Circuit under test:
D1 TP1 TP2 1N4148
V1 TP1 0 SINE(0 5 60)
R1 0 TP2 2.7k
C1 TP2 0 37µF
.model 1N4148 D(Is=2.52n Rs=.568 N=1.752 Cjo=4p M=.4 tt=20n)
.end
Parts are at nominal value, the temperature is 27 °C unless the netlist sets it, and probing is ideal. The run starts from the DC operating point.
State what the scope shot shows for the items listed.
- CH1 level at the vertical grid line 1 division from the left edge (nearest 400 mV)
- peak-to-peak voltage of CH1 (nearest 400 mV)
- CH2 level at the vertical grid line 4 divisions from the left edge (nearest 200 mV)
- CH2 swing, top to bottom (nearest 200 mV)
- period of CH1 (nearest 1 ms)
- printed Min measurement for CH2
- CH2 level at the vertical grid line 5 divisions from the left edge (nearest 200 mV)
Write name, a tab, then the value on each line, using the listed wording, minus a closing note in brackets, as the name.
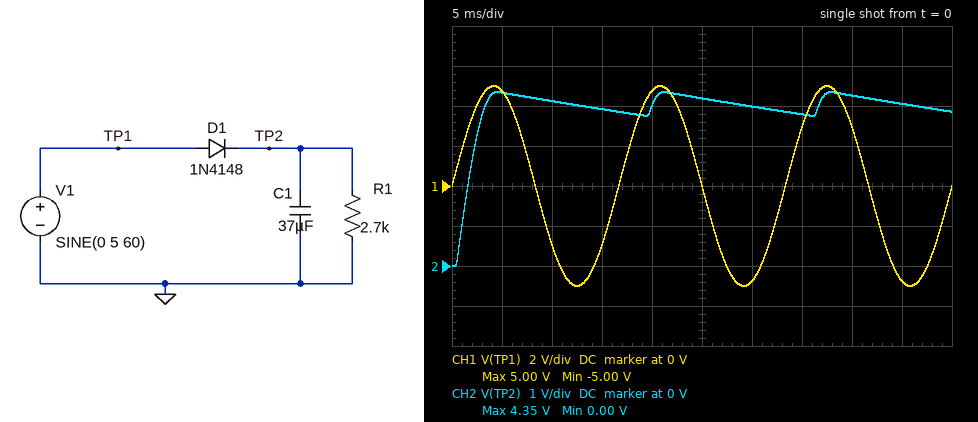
CH1 level at the vertical grid line 1 division from the left edge	4.8 V
peak-to-peak voltage of CH1	10.0 V
CH2 level at the vertical grid line 4 divisions from the left edge	4.0 V
CH2 swing, top to bottom	4.4 V
period of CH1	17 ms
printed Min measurement for CH2	0.00 V
CH2 level at the vertical grid line 5 divisions from the left edge	4.2 V
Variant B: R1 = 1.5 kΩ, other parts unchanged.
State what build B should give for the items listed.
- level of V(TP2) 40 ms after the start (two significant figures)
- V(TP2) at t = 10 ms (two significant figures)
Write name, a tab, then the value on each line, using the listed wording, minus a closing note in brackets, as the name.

level of V(TP2) 40 ms after the start	4.2 V
V(TP2) at t = 10 ms	3.9 V
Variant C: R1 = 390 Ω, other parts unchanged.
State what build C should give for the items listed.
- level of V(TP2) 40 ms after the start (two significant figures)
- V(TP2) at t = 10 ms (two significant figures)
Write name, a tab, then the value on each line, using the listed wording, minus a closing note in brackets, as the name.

level of V(TP2) 40 ms after the start	3.7 V
V(TP2) at t = 10 ms	3.0 V
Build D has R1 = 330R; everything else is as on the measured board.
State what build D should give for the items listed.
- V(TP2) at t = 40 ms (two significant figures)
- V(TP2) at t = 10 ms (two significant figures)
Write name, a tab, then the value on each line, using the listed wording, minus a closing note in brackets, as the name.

V(TP2) at t = 40 ms	3.6 V
V(TP2) at t = 10 ms	2.8 V
